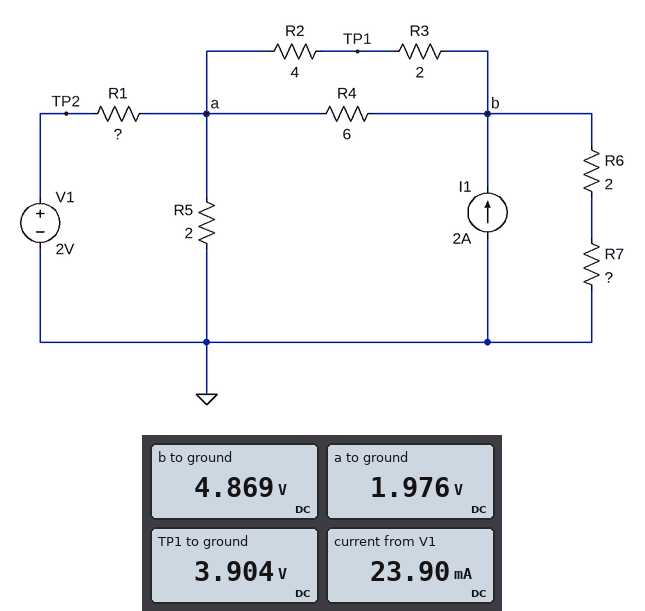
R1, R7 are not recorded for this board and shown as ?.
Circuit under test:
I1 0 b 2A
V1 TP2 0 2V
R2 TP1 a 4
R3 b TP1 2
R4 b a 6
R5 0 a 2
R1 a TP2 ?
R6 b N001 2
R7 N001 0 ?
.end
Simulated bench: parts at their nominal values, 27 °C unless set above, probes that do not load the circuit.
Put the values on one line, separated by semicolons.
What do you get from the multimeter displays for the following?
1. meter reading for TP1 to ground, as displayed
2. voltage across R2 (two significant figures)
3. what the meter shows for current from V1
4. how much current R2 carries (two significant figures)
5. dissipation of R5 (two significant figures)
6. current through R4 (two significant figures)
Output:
3.904 V; 1.9 V; 23.90 mA; 480 mA; 2.0 W; 480 mA
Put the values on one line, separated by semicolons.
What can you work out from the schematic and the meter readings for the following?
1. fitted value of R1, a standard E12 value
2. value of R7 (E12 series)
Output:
1 Ω; 2.7 Ω
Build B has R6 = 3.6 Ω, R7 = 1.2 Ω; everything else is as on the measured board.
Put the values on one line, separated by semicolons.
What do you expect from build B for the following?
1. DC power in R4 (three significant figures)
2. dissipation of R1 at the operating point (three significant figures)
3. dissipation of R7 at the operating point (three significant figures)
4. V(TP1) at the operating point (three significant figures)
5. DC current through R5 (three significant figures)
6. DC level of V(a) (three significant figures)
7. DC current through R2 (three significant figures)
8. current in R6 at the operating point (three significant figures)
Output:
1.43 W; 248 µW; 1.26 W; 3.94 V; 992 mA; 1.98 V; 488 mA; 1.02 A
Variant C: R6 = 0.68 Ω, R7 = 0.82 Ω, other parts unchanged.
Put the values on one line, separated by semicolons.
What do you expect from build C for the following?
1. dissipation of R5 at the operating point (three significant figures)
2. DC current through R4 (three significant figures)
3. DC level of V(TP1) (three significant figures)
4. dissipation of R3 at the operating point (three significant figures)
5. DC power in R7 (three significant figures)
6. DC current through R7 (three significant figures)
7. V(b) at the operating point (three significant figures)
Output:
1.20 W; 161 mA; 2.19 V; 52.0 mW; 2.31 W; 1.68 A; 2.52 V
